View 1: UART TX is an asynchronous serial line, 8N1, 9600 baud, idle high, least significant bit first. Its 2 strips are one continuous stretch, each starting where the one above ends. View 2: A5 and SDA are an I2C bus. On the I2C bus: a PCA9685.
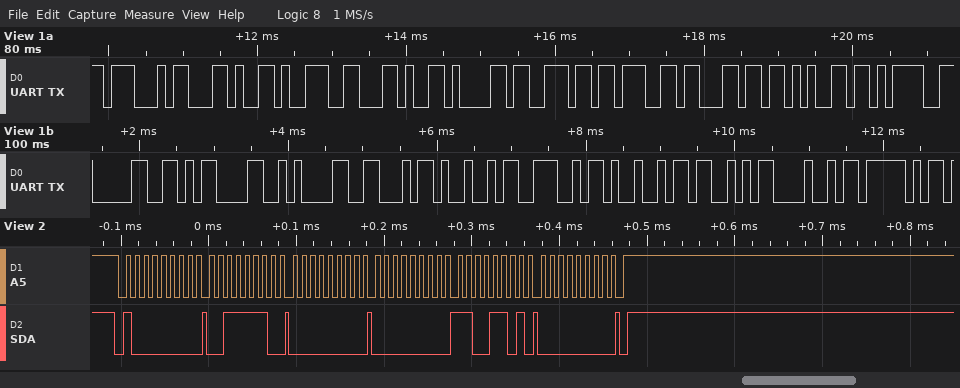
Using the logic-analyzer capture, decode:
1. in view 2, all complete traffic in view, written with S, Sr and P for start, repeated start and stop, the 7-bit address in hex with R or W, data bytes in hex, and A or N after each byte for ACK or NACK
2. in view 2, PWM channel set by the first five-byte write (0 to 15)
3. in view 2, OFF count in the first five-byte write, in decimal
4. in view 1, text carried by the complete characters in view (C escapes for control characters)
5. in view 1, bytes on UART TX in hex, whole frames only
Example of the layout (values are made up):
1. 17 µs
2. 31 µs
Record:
1. S 40W A 3E A 00 A 00 A CD A 00 A P
2. 14
3. 205
4. "G,9,angle=0\r\nFINISH_"
5. 0x47 0x2C 0x39 0x2C 0x61 0x6E 0x67 0x6C 0x65 0x3D 0x30 0x0D 0x0A 0x46 0x49 0x4E 0x49 0x53 0x48 0x5F
